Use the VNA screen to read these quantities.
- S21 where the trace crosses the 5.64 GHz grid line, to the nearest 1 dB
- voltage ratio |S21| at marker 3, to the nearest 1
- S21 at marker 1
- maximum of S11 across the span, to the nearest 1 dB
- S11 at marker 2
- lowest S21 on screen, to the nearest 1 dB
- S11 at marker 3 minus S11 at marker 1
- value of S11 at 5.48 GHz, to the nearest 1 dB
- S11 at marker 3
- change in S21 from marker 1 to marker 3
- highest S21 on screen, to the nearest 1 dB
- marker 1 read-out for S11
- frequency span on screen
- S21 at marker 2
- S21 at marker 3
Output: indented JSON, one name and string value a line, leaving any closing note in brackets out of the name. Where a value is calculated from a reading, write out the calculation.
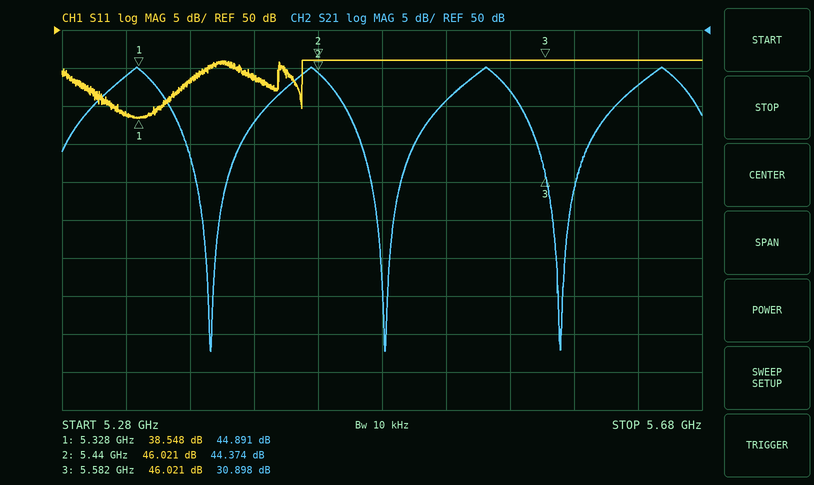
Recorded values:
{
  "S21 where the trace crosses the 5.64 GHz grid line, to the nearest 1 dB": "43 dB",
  "voltage ratio |S21| at marker 3, to the nearest 1": "10^(30.898/20) ≈ 35",
  "S21 at marker 1": "44.891 dB",
  "maximum of S11 across the span, to the nearest 1 dB": "46 dB",
  "S11 at marker 2": "46.021 dB",
  "lowest S21 on screen, to the nearest 1 dB": "8 dB",
  "S11 at marker 3 minus S11 at marker 1": "46.021 − (38.548) = 7.473 dB",
  "value of S11 at 5.48 GHz, to the nearest 1 dB": "46 dB",
  "S11 at marker 3": "46.021 dB",
  "change in S21 from marker 1 to marker 3": "30.898 − (44.891) = -13.993 dB",
  "highest S21 on screen, to the nearest 1 dB": "45 dB",
  "marker 1 read-out for S11": "38.548 dB",
  "frequency span on screen": "400 MHz",
  "S21 at marker 2": "44.374 dB",
  "S21 at marker 3": "30.898 dB"
}
